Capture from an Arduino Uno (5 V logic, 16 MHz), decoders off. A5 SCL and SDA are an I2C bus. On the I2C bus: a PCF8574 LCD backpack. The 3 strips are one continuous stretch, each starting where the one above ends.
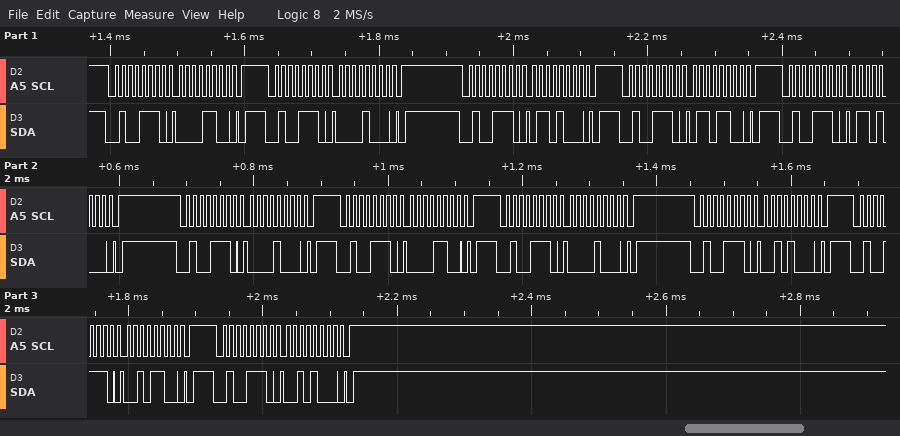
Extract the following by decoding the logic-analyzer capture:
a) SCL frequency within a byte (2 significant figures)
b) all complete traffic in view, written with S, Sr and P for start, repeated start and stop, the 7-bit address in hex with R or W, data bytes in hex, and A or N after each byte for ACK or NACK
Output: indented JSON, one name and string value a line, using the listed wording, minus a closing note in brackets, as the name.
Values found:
{
  "SCL frequency within a byte": "100 kHz",
  "all complete traffic in view, written with S, Sr and P for start, repeated start and stop, the 7-bit address in hex with R or W, data bytes in hex, and A or N after each byte for ACK or NACK": "S 27W A 0C A P S 27W A 08 A P S 27W A 68 A P S 27W A 6C A P S 27W A 68 A P S 27W A 08 A P S 27W A 0C A P S 27W A 08 A P S 27W A 28 A P S 27W A 2C A P S 27W A 28 A P"
}
